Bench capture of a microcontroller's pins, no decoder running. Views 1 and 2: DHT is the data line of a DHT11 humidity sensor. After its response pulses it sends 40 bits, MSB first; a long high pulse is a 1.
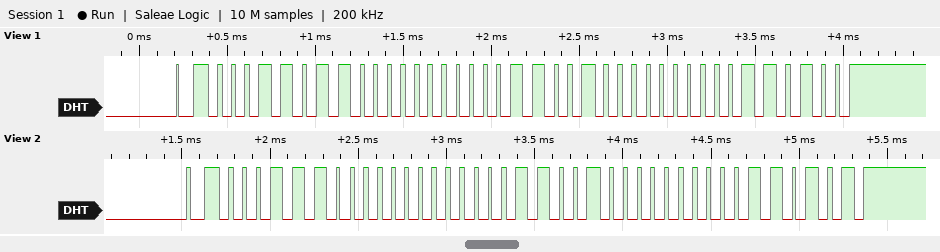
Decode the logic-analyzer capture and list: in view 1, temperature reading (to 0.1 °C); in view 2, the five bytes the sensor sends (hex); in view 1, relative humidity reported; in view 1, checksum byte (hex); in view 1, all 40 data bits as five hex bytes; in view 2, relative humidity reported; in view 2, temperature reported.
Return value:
25.0 °C
1C 00 19 00 35
27 %
0x34
1B 00 19 00 34
28 %
25.0 °C
